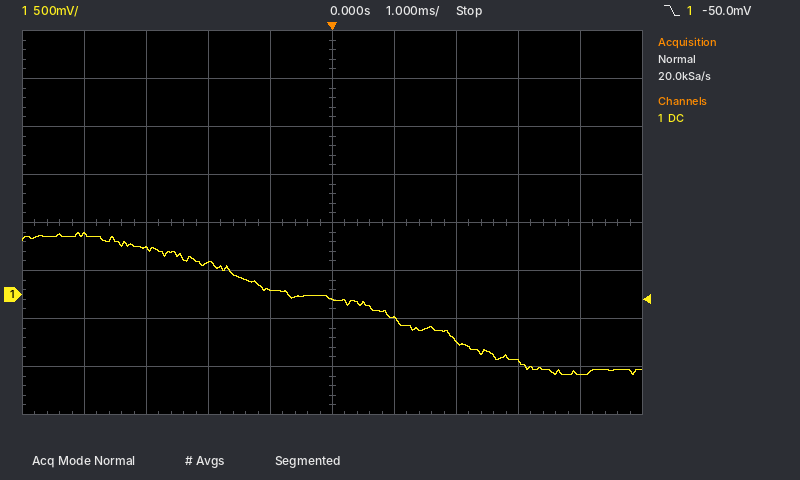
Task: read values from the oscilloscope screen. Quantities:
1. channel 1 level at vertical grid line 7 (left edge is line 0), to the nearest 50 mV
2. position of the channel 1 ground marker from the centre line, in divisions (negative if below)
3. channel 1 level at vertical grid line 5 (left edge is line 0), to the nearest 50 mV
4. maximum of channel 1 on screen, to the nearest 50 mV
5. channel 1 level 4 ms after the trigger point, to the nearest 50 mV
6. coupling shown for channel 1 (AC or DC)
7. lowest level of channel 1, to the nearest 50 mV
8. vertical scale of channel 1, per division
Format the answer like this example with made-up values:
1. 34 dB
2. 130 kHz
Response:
1. -500 mV
2. -1.5 div
3. -50 mV
4. 650 mV
5. -850 mV
6. DC
7. -850 mV
8. 500 mV
